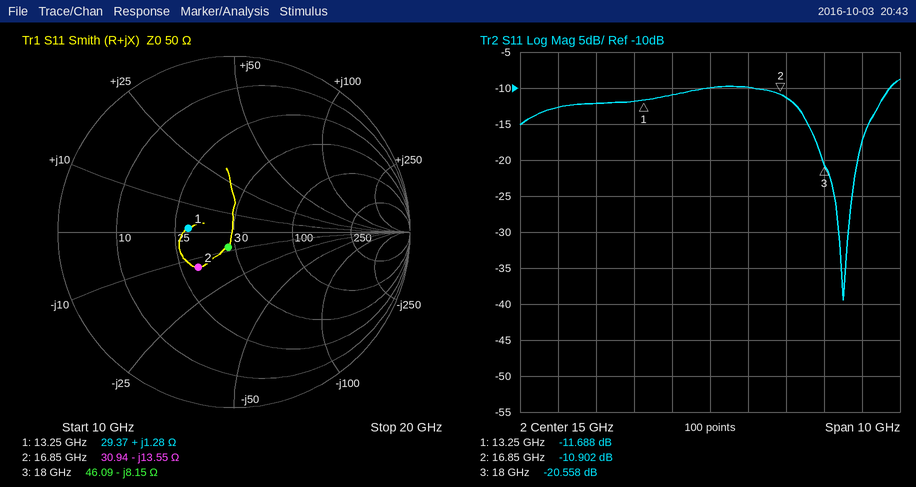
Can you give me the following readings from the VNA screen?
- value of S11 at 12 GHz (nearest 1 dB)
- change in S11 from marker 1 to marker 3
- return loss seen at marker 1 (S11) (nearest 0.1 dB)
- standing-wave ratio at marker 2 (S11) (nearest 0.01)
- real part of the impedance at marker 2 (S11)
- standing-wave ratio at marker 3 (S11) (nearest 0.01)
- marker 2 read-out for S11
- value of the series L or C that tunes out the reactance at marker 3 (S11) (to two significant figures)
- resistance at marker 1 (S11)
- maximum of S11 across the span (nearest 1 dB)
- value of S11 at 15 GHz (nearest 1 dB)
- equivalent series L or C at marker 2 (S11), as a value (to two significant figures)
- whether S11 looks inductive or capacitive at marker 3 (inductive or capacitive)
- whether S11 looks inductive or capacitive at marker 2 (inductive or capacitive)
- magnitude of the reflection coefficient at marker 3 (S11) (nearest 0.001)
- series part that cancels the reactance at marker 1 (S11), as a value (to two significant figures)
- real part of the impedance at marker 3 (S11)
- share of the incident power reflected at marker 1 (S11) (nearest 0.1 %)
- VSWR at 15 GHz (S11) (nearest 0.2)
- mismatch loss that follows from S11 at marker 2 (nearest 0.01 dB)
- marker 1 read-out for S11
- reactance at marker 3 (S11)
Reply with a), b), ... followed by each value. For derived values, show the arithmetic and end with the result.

a) -12 dB
b) -20.558 − (-11.688) = -8.870 dB
c) 11.7 dB
d) 1.80
e) 30.94 Ω
f) 1.21
g) -10.902 dB
h) L = 8.15 Ω/(2π × 18 GHz) ≈ 72 pH
i) 29.37 Ω
j) -9 dB
k) -10 dB
l) C = 1/(2π × 16.85 GHz × 13.55 Ω) ≈ 697 fF, so 700 fF to two significant figures
m) capacitive
n) capacitive
o) 10^(-20.558/20) ≈ 0.094
p) C = 1/(2π × 13.25 GHz × 1.28 Ω) ≈ 9.4 pF
q) 46.09 Ω
r) 10^(-11.688/10) ≈ 6.8 %
s) |Γ| = 10^(-10/20) = 0.3162; VSWR = (1 + 0.3162)/(1 − 0.3162) ≈ 1.92, so 2.0 to the nearest 0.2
t) −10 log10(1 − 10^(-10.902/10)) ≈ 0.37 dB
u) -11.688 dB
v) -8.15 Ω
